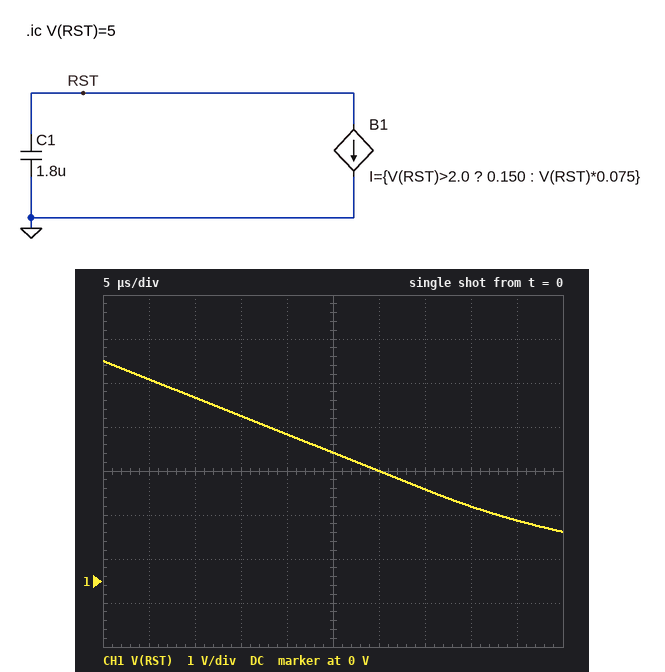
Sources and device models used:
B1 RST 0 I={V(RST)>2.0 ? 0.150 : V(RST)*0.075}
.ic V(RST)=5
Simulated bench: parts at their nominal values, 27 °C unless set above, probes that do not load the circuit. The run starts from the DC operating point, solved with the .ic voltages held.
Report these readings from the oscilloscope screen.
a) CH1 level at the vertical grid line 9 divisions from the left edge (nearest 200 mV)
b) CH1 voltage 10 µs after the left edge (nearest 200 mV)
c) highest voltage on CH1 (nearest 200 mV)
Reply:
1.4 V
4.2 V
5.0 V
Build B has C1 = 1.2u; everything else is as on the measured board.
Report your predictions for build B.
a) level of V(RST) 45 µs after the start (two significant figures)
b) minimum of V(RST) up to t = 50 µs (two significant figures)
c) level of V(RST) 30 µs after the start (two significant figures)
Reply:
540 mV
390 mV
1.4 V
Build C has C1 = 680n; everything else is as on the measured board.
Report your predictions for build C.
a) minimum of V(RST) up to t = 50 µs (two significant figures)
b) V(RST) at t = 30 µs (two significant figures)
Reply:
36 mV
330 mV
